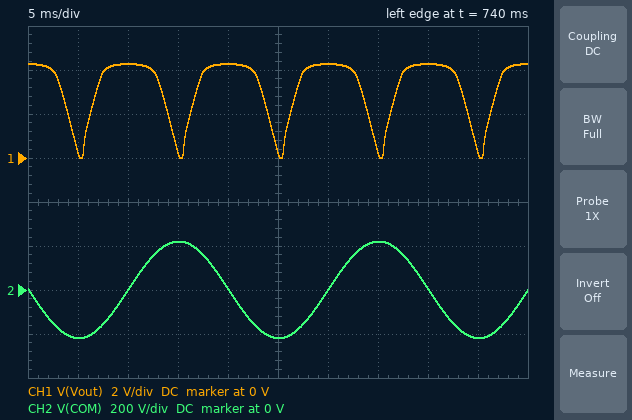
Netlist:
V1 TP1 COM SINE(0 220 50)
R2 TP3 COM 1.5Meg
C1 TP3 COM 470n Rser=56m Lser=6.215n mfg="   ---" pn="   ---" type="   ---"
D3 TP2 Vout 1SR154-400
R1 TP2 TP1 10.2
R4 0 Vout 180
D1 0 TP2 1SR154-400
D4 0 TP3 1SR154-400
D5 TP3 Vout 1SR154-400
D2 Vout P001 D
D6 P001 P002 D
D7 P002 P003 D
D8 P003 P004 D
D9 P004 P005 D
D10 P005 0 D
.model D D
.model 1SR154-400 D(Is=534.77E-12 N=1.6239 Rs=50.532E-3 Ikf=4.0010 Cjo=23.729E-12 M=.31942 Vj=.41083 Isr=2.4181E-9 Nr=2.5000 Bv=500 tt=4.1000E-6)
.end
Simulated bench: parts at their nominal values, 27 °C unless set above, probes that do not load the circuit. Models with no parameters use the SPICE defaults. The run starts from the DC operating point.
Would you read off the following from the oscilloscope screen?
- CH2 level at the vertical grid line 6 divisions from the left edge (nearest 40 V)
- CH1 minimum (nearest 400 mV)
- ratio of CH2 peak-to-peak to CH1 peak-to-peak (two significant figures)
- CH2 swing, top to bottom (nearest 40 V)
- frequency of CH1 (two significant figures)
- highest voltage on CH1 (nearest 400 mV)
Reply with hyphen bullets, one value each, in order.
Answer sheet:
- 0 V
- 0 V
- 100
- 440 V
- 100 Hz
- 4.4 V
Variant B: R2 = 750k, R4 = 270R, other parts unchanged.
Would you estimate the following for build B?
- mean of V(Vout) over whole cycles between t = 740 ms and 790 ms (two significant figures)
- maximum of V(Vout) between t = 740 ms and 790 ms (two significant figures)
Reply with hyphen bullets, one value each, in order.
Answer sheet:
- 3.6 V
- 4.4 V
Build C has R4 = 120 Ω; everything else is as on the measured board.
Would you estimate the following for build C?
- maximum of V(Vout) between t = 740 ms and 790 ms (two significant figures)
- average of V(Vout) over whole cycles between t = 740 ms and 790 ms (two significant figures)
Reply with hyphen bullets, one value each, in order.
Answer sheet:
- 3.8 V
- 2.5 V
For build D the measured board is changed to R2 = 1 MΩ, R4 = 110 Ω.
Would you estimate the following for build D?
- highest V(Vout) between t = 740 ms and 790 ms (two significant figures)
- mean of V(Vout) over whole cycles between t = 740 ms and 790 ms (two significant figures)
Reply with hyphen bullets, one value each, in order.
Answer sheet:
- 3.6 V
- 2.3 V
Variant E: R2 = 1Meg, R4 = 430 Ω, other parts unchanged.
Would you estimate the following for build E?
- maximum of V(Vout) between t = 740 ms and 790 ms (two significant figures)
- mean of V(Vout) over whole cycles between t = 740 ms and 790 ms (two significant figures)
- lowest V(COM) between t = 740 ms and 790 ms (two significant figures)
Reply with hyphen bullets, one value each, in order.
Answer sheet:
- 4.4 V
- 3.8 V
- -220 V
